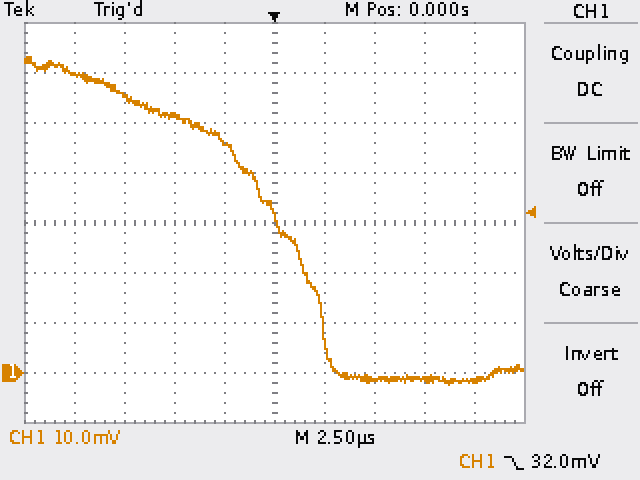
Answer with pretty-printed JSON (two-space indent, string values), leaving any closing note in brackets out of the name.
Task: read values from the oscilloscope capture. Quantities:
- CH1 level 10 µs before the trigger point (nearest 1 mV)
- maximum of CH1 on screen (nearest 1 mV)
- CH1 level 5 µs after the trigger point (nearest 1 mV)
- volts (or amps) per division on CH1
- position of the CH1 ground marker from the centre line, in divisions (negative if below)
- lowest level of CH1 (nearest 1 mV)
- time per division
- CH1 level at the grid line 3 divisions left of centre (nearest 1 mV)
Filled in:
{
  "CH1 level 10 µs before the trigger point": "60 mV",
  "maximum of CH1 on screen": "63 mV",
  "CH1 level 5 µs after the trigger point": "-1 mV",
  "volts (or amps) per division on CH1": "10 mV",
  "position of the CH1 ground marker from the centre line, in divisions": "-3.0 div",
  "lowest level of CH1": "-2 mV",
  "time per division": "2.5 µs",
  "CH1 level at the grid line 3 divisions left of centre": "55 mV"
}
